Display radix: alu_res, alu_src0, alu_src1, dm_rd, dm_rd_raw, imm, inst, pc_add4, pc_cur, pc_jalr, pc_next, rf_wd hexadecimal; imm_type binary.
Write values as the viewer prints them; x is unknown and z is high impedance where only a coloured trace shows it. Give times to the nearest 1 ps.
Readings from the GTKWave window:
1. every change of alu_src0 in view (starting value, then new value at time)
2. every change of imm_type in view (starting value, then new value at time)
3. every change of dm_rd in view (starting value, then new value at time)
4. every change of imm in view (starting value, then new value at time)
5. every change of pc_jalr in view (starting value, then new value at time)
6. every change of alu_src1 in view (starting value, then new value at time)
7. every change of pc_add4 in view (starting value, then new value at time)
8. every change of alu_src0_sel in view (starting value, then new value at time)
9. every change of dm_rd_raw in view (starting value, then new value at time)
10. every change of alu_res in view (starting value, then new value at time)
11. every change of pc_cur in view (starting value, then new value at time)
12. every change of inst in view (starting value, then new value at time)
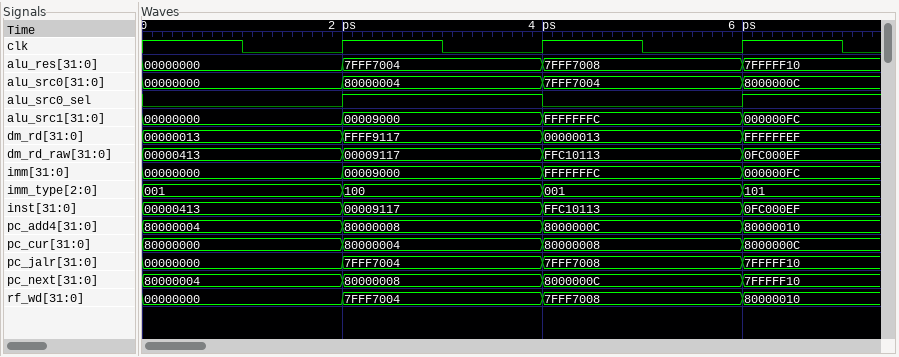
00000000, 80000004 at 2 ps, 7FFF7004 at 4 ps, 8000000C at 6 ps
001, 100 at 2 ps, 001 at 4 ps, 101 at 6 ps
00000013, FFFF9117 at 2 ps, 00000013 at 4 ps, FFFFFFEF at 6 ps
00000000, 00009000 at 2 ps, FFFFFFFC at 4 ps, 000000FC at 6 ps
00000000, 7FFF7004 at 2 ps, 7FFF7008 at 4 ps, 7FFFFF10 at 6 ps
00000000, 00009000 at 2 ps, FFFFFFFC at 4 ps, 000000FC at 6 ps
80000004, 80000008 at 2 ps, 8000000C at 4 ps, 80000010 at 6 ps
0, 1 at 2 ps, 0 at 4 ps, 1 at 6 ps
00000413, 00009117 at 2 ps, FFC10113 at 4 ps, 0FC000EF at 6 ps
00000000, 7FFF7004 at 2 ps, 7FFF7008 at 4 ps, 7FFFFF10 at 6 ps
80000000, 80000004 at 2 ps, 80000008 at 4 ps, 8000000C at 6 ps
00000413, 00009117 at 2 ps, FFC10113 at 4 ps, 0FC000EF at 6 ps
